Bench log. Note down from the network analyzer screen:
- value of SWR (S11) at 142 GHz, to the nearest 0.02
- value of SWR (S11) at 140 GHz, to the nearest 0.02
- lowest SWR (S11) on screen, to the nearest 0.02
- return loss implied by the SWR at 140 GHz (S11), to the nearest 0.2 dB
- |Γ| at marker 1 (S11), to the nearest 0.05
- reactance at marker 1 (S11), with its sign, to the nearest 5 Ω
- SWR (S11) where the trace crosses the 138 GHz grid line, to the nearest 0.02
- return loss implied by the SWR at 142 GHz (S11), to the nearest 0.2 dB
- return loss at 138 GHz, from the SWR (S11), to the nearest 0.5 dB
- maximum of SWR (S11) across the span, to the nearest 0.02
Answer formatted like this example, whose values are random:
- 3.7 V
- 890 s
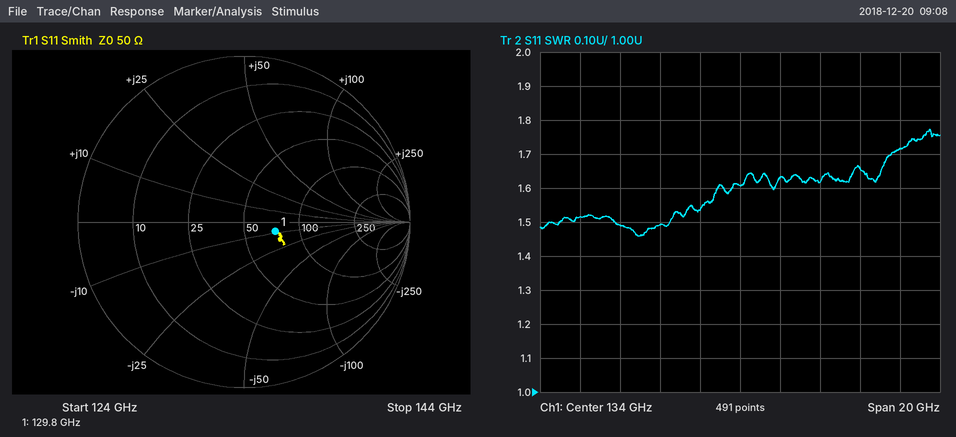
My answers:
- 1.72
- 1.66
- 1.46
- 12.2 dB
- 0.20
- -10 Ω
- 1.62
- 11.6 dB
- 12.5 dB
- 1.78
